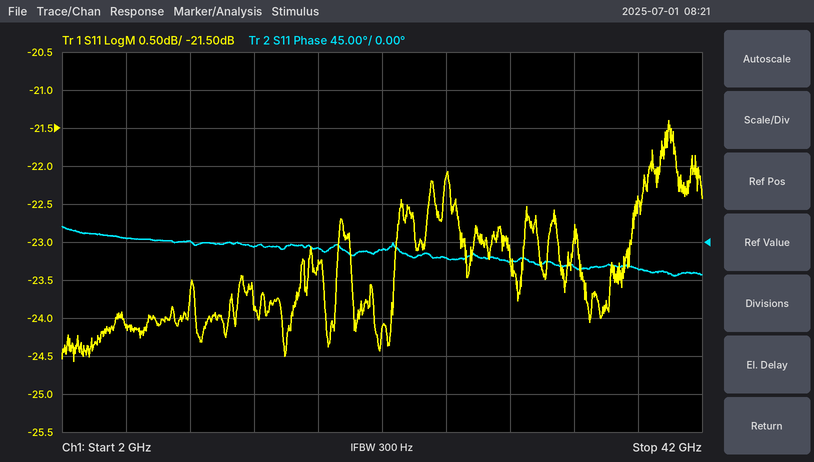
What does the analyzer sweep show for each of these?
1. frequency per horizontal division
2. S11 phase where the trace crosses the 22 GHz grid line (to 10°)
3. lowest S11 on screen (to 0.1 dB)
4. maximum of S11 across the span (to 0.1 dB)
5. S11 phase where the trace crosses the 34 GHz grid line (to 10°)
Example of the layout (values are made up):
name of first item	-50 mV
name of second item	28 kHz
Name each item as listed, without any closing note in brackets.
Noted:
frequency per horizontal division	4 GHz
S11 phase where the trace crosses the 22 GHz grid line	-10°
lowest S11 on screen	-24.6 dB
maximum of S11 across the span	-21.4 dB
S11 phase where the trace crosses the 34 GHz grid line	-30°
